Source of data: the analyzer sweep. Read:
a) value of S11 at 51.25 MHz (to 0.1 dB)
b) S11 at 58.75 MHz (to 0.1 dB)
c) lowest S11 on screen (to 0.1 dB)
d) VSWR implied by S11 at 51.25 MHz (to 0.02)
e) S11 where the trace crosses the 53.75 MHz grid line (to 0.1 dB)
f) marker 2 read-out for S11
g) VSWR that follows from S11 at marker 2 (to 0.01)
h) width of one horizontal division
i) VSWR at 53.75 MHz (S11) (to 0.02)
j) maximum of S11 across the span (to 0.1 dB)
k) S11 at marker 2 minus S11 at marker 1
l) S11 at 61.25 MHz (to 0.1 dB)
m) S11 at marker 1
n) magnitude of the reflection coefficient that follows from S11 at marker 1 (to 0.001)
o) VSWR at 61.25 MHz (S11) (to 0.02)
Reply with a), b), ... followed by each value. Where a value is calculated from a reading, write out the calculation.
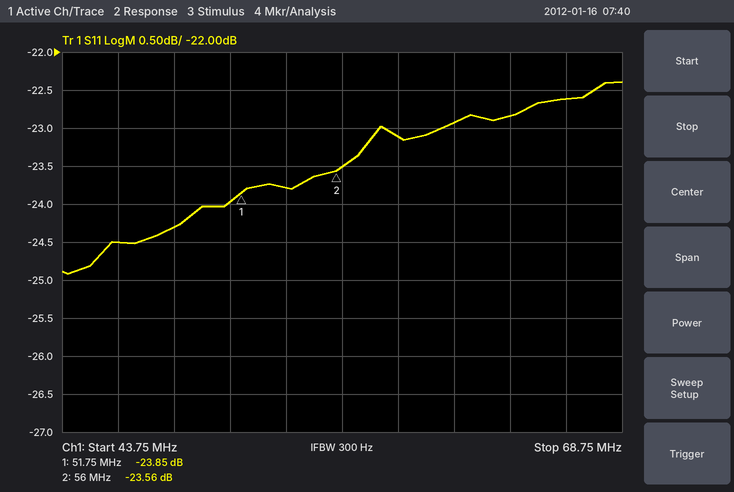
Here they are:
a) -24.0 dB
b) -23.1 dB
c) -24.9 dB
d) |Γ| = 10^(-24/20) = 0.0631; VSWR = (1 + 0.0631)/(1 − 0.0631) ≈ 1.13, so 1.14 to the nearest 0.02
e) -23.8 dB
f) -23.56 dB
g) (1 + 0.0664)/(1 − 0.0664) ≈ 1.14
h) 2.5 MHz
i) |Γ| = 10^(-23.8/20) = 0.0646; VSWR = (1 + 0.0646)/(1 − 0.0646) ≈ 1.14
j) -22.4 dB
k) -23.56 − (-23.85) = 0.29 dB
l) -22.9 dB
m) -23.85 dB
n) 10^(-23.85/20) ≈ 0.064
o) |Γ| = 10^(-22.9/20) = 0.0716; VSWR = (1 + 0.0716)/(1 − 0.0716) ≈ 1.15, so 1.16 to the nearest 0.02
